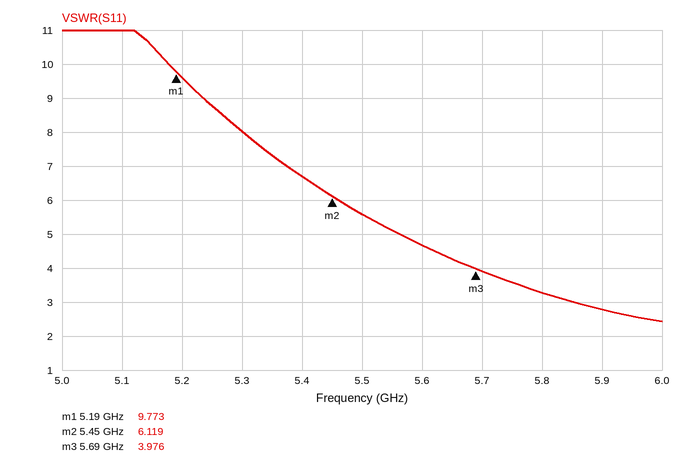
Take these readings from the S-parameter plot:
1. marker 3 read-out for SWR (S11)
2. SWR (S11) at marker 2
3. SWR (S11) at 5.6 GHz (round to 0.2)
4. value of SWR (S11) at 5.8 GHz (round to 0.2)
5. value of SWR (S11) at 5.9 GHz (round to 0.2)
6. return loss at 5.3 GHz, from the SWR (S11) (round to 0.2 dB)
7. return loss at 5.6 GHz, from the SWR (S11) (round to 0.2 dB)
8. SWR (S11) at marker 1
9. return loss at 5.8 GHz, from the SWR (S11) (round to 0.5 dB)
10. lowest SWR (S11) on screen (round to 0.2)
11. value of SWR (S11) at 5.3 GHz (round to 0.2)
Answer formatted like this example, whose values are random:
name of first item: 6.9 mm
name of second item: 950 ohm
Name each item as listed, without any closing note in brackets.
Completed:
marker 3 read-out for SWR: 3.976
SWR (S11) at marker 2: 6.119
SWR (S11) at 5.6 GHz: 4.6
value of SWR (S11) at 5.8 GHz: 3.2
value of SWR (S11) at 5.9 GHz: 2.8
return loss at 5.3 GHz, from the SWR (S11): 2.2 dB
return loss at 5.6 GHz, from the SWR (S11): 3.8 dB
SWR (S11) at marker 1: 9.773
return loss at 5.8 GHz, from the SWR (S11): 5.5 dB
lowest SWR (S11) on screen: 2.4
value of SWR (S11) at 5.3 GHz: 8.0
